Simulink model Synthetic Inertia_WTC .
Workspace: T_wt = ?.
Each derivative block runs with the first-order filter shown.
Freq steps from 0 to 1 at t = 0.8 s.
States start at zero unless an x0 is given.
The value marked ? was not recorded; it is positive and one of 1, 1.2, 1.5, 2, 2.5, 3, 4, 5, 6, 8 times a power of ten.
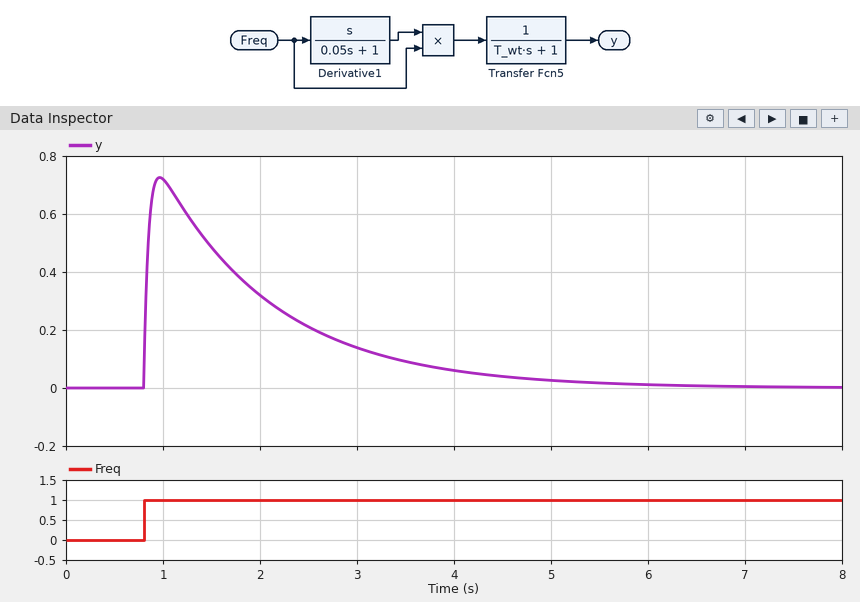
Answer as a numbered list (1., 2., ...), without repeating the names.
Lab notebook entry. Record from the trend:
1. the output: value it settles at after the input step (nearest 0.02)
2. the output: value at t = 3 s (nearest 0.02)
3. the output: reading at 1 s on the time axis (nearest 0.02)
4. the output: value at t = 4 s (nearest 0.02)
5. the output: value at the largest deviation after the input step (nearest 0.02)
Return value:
1. 0.00
2. 0.14
3. 0.72
4. 0.06
5. 0.72
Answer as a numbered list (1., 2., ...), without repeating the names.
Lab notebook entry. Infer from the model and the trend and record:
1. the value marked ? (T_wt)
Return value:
1. 1.2
